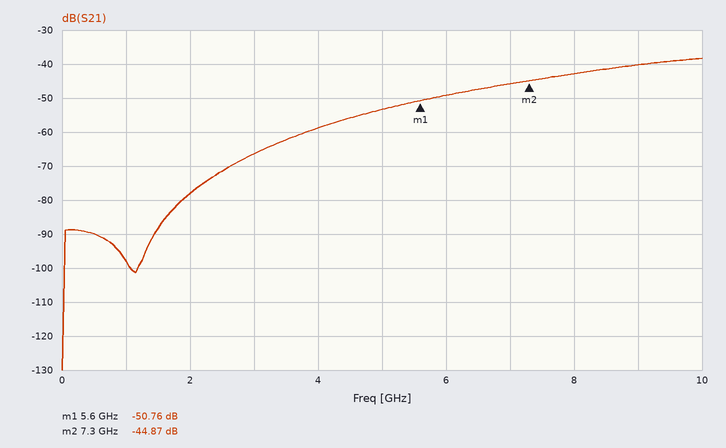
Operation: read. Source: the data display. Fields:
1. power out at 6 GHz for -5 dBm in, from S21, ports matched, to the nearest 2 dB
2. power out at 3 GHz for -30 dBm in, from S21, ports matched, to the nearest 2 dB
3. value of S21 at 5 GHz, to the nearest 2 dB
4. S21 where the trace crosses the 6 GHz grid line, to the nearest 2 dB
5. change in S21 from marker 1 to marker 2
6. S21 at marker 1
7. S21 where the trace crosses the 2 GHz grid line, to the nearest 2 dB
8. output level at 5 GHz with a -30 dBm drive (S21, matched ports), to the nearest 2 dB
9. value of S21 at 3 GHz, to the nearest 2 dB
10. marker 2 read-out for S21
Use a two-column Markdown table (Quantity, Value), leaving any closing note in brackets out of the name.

| Quantity | Value |
|---|---|
| power out at 6 GHz for -5 dBm in, from S21, ports matched, to the nearest 2 dB | -54 dBm |
| power out at 3 GHz for -30 dBm in, from S21, ports matched, to the nearest 2 dB | -96 dBm |
| value of S21 at 5 GHz, to the nearest 2 dB | -54 dB |
| S21 where the trace crosses the 6 GHz grid line, to the nearest 2 dB | -50 dB |
| change in S21 from marker 1 to marker 2 | 5.89 dB |
| S21 at marker 1 | -50.76 dB |
| S21 where the trace crosses the 2 GHz grid line, to the nearest 2 dB | -78 dB |
| output level at 5 GHz with a -30 dBm drive (S21, matched ports), to the nearest 2 dB | -84 dBm |
| value of S21 at 3 GHz, to the nearest 2 dB | -66 dB |
| marker 2 read-out for S21 | -44.87 dB |
